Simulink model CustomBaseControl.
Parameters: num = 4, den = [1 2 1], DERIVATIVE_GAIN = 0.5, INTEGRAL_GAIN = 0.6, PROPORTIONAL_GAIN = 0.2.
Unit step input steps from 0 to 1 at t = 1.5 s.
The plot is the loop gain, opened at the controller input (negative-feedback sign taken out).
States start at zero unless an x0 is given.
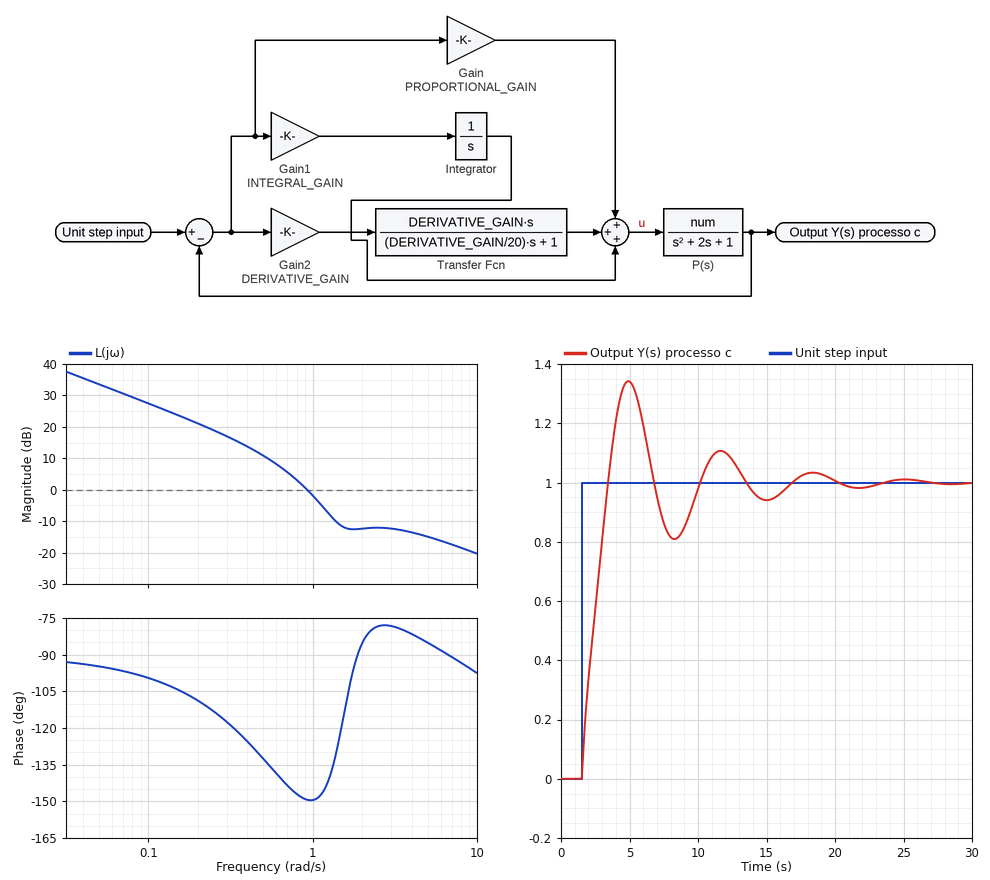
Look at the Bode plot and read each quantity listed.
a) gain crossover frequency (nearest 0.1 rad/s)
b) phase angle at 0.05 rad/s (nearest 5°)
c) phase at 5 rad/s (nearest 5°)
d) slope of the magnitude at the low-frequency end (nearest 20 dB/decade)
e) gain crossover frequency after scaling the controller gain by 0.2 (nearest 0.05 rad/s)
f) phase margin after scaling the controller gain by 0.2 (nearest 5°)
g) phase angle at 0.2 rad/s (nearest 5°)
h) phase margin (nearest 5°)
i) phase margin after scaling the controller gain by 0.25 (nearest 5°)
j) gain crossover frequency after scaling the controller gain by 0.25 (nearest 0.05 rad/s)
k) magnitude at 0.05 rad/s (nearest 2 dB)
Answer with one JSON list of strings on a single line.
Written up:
["0.9 rad/s", "-95°", "-85°", "-20 dB/decade", "0.40 rad/s", "55°", "-110°", "30°", "50°", "0.45 rad/s", "34 dB"]
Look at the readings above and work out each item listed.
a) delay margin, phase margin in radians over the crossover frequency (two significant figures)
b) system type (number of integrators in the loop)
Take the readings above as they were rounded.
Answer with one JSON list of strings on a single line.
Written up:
["0.58 s", "1"]
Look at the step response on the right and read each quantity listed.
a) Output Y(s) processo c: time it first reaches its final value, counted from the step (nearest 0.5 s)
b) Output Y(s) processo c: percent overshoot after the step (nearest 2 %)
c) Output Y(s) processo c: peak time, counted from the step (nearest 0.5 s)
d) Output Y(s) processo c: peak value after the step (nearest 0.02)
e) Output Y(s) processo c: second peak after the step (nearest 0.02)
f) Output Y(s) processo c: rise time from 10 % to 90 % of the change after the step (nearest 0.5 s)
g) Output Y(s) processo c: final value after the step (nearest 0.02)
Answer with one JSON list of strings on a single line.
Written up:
["2.0 s", "34 %", "3.5 s", "1.34", "1.10", "1.5 s", "1.00"]
